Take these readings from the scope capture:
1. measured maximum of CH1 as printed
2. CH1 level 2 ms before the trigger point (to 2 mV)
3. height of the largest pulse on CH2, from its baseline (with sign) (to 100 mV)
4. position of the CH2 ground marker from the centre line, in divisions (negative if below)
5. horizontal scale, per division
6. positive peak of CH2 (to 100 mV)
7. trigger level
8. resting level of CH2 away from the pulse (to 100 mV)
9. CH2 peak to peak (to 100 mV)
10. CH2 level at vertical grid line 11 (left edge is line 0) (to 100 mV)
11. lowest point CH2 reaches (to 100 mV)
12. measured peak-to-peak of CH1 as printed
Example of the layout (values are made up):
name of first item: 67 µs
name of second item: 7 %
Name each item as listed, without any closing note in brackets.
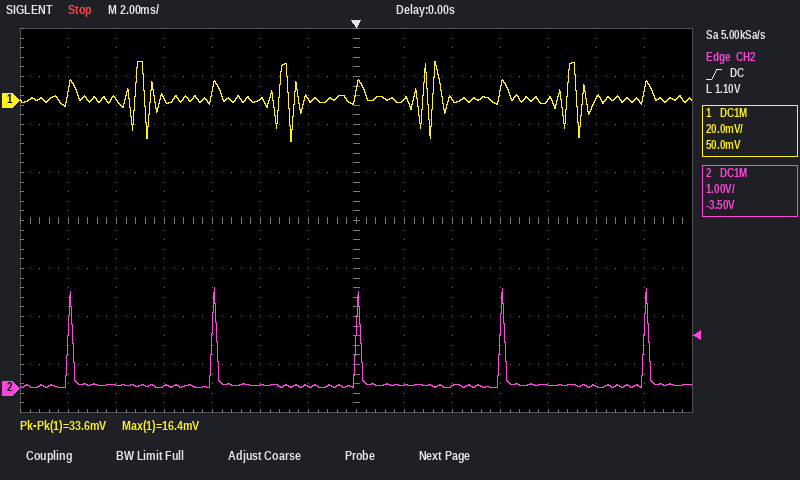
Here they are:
measured maximum of CH1 as printed: 16.4 mV
CH1 level 2 ms before the trigger point: 0 mV
height of the largest pulse on CH2, from its baseline (with sign): +2.0 V
position of the CH2 ground marker from the centre line, in divisions: -3.5 div
horizontal scale, per division: 2 ms
positive peak of CH2: 2.1 V
trigger level: 1.10 V
resting level of CH2 away from the pulse: 100 mV
CH2 peak to peak: 2.1 V
CH2 level at vertical grid line 11 (left edge is line 0): 100 mV
lowest point CH2 reaches: 0.0 V
measured peak-to-peak of CH1 as printed: 33.6 mV
